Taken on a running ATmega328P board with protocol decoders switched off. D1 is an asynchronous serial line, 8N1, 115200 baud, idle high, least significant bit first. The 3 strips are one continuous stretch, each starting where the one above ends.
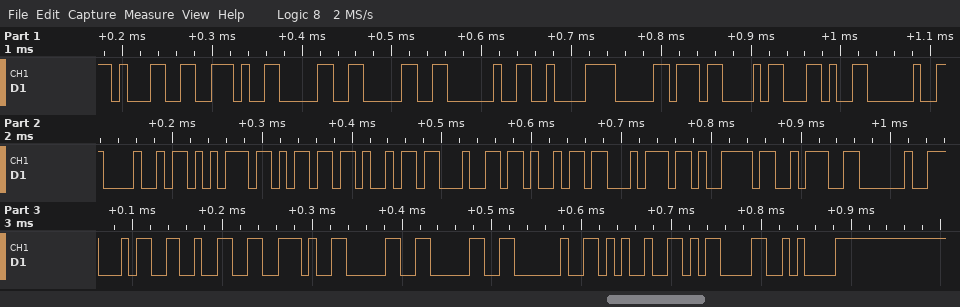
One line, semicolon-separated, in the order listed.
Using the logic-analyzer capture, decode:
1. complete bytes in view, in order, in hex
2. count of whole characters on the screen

0x31 0x2E 0x30 0x30 0x20 0xC2 0xB0 0x43 0x2C 0x20 0x48 0x75 0x6D 0x69 0x64 0x69 0x74 0x79 0x3A 0x20 0x34 0x32 0x2E 0x30 0x30 0x20 0x25 0x0D 0x0A; 29
